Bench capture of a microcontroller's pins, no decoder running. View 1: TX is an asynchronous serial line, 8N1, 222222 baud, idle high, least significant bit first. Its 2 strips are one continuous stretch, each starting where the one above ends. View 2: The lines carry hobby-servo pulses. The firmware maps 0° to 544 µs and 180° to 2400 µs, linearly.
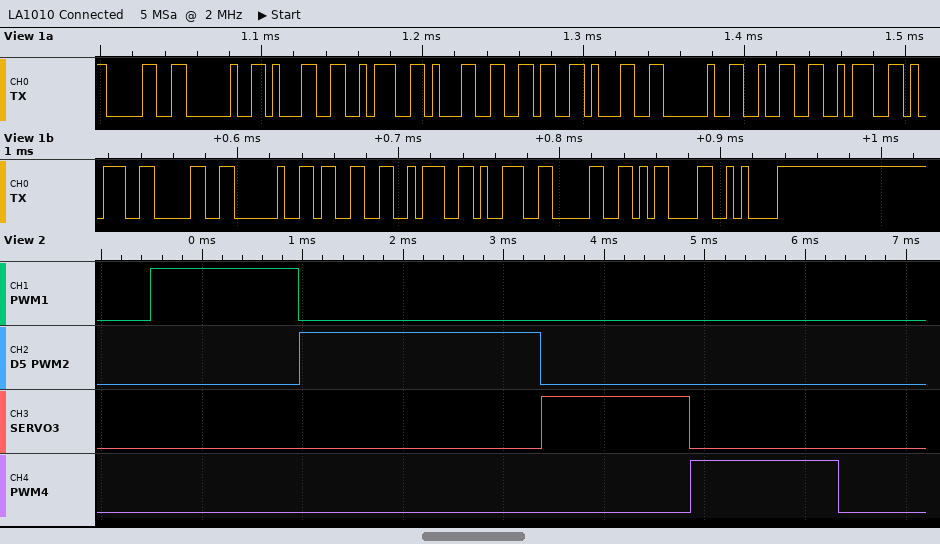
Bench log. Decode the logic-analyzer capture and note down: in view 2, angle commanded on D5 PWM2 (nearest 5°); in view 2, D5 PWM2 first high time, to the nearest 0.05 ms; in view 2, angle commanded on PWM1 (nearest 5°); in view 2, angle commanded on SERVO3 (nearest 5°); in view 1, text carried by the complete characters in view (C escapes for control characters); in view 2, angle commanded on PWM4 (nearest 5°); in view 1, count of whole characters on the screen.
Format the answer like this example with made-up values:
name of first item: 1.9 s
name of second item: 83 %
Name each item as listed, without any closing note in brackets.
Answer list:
in view 2, angle commanded on D5 PWM2: 180°
in view 2, D5 PWM2 first high time, to the nearest 0.05 ms: 2.40 ms
in view 2, angle commanded on PWM1: 90°
in view 2, angle commanded on SERVO3: 90°
in view 1, text carried by the complete characters in view: "0 1:161 2:90 3:90\r\n"
in view 2, angle commanded on PWM4: 90°
in view 1, count of whole characters on the screen: 19
